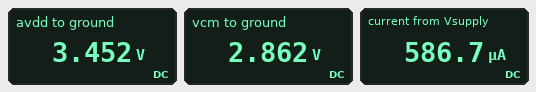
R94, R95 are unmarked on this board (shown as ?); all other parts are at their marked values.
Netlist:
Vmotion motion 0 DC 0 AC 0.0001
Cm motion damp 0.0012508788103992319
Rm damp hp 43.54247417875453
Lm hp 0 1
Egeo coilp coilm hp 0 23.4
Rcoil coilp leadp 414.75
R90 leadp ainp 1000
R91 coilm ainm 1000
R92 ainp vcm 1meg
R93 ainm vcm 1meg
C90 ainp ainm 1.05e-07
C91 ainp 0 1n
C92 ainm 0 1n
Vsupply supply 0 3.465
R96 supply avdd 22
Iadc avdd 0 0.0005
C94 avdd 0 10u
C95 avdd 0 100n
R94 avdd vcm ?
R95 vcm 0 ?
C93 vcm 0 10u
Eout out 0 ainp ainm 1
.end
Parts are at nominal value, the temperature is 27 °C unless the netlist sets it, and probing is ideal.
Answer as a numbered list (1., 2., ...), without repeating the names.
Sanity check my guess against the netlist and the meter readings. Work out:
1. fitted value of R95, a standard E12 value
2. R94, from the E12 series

1. 33 kΩ
2. 6.8 kΩ
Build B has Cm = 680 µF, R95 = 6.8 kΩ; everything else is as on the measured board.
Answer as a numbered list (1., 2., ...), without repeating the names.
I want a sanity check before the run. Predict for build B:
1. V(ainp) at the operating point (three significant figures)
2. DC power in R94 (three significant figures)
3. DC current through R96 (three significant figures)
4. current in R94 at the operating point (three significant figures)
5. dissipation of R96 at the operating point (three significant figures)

1. 1.72 V
2. 437 µW
3. 754 µA
4. 254 µA
5. 12.5 µW
